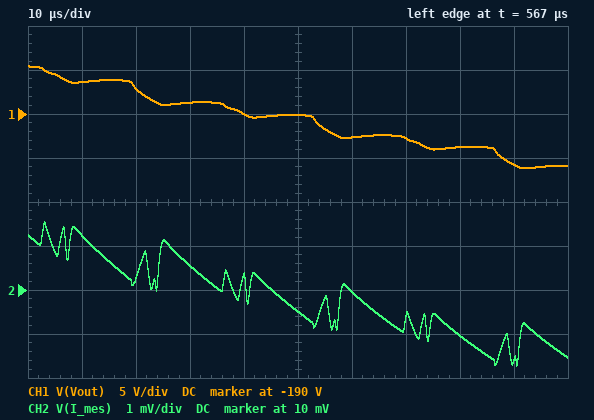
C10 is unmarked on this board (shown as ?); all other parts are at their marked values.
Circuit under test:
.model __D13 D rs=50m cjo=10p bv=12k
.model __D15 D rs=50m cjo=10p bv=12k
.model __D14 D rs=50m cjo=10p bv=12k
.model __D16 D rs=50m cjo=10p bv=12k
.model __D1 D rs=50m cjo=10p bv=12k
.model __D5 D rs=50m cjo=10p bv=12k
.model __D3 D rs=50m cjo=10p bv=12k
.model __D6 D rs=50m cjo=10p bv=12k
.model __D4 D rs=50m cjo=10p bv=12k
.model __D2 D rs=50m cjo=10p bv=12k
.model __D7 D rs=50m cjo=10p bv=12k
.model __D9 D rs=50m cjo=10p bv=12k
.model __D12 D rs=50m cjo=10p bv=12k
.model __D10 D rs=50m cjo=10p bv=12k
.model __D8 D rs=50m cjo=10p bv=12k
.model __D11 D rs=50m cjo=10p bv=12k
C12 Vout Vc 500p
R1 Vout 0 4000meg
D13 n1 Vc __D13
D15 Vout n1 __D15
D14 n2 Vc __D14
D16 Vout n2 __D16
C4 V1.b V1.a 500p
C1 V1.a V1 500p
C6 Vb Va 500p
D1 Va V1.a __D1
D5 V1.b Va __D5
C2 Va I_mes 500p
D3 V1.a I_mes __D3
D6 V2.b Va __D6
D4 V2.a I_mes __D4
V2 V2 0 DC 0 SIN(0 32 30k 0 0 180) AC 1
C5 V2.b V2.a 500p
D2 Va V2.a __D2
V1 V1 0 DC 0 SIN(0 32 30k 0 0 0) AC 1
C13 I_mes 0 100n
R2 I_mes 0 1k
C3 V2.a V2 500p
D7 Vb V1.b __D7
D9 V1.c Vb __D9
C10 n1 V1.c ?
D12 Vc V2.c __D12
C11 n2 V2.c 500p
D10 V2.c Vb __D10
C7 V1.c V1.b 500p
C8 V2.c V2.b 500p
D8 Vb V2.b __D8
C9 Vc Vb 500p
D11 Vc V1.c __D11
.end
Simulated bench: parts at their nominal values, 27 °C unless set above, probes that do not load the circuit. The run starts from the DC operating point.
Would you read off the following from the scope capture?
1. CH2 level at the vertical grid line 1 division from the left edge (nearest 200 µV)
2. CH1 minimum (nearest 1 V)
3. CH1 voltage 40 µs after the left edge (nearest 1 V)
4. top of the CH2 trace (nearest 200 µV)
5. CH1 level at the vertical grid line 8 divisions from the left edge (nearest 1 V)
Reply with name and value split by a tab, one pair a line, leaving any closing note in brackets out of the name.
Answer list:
CH2 level at the vertical grid line 1 division from the left edge	11.2 mV
CH1 minimum	-196 V
CH1 voltage 40 µs after the left edge	-190 V
top of the CH2 trace	11.6 mV
CH1 level at the vertical grid line 8 divisions from the left edge	-194 V
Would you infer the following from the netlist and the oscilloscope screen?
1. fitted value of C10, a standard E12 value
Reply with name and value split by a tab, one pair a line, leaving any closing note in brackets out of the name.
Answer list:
fitted value of C10, a standard E12 value	1.2 nF
